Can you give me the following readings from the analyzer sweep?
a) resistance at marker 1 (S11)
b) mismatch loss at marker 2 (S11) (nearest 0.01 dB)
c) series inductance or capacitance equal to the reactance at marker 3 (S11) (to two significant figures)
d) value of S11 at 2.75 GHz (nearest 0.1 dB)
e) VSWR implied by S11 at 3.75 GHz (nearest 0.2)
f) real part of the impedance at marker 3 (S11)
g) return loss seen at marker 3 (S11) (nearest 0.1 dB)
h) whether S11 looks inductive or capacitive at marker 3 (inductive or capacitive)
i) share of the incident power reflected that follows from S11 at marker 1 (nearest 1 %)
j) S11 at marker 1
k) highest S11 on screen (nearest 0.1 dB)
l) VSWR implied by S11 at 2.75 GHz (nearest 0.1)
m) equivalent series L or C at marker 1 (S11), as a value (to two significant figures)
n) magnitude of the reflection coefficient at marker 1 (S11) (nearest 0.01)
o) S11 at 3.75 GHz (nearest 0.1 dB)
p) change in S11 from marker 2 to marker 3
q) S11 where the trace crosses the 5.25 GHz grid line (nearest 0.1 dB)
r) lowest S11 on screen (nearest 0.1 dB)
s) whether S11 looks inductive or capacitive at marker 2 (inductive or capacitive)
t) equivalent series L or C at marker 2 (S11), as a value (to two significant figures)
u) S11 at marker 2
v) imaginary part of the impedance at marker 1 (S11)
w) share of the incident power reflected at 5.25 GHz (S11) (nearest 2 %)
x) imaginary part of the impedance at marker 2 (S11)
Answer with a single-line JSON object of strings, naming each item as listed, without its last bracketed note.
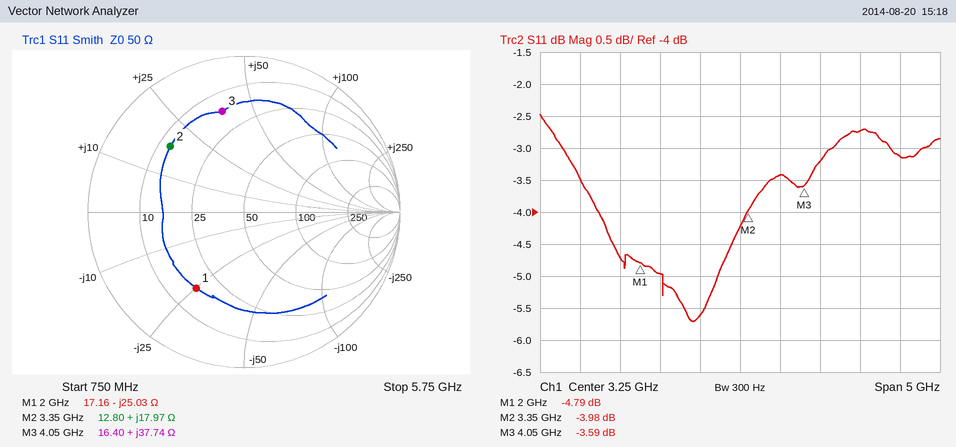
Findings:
{"resistance at marker 1": "17.16 Ω", "mismatch loss at marker 2 (S11)": "2.22 dB", "series inductance or capacitance equal to the reactance at marker 3 (S11)": "1.5 nH", "value of S11 at 2.75 GHz": "-5.6 dB", "VSWR implied by S11 at 3.75 GHz": "5.2", "real part of the impedance at marker 3": "16.40 Ω", "return loss seen at marker 3 (S11)": "3.6 dB", "whether S11 looks inductive or capacitive at marker 3": "inductive", "share of the incident power reflected that follows from S11 at marker 1": "33 %", "S11 at marker 1": "-4.79 dB", "highest S11 on screen": "-2.5 dB", "VSWR implied by S11 at 2.75 GHz": "3.2", "equivalent series L or C at marker 1 (S11), as a value": "3.2 pF", "magnitude of the reflection coefficient at marker 1 (S11)": "0.58", "S11 at 3.75 GHz": "-3.4 dB", "change in S11 from marker 2 to marker 3": "0.39 dB", "S11 where the trace crosses the 5.25 GHz grid line": "-3.1 dB", "lowest S11 on screen": "-5.7 dB", "whether S11 looks inductive or capacitive at marker 2": "inductive", "equivalent series L or C at marker 2 (S11), as a value": "850 pH", "S11 at marker 2": "-3.98 dB", "imaginary part of the impedance at marker 1": "-25.03 Ω", "share of the incident power reflected at 5.25 GHz (S11)": "48 %", "imaginary part of the impedance at marker 2": "+17.97 Ω"}
